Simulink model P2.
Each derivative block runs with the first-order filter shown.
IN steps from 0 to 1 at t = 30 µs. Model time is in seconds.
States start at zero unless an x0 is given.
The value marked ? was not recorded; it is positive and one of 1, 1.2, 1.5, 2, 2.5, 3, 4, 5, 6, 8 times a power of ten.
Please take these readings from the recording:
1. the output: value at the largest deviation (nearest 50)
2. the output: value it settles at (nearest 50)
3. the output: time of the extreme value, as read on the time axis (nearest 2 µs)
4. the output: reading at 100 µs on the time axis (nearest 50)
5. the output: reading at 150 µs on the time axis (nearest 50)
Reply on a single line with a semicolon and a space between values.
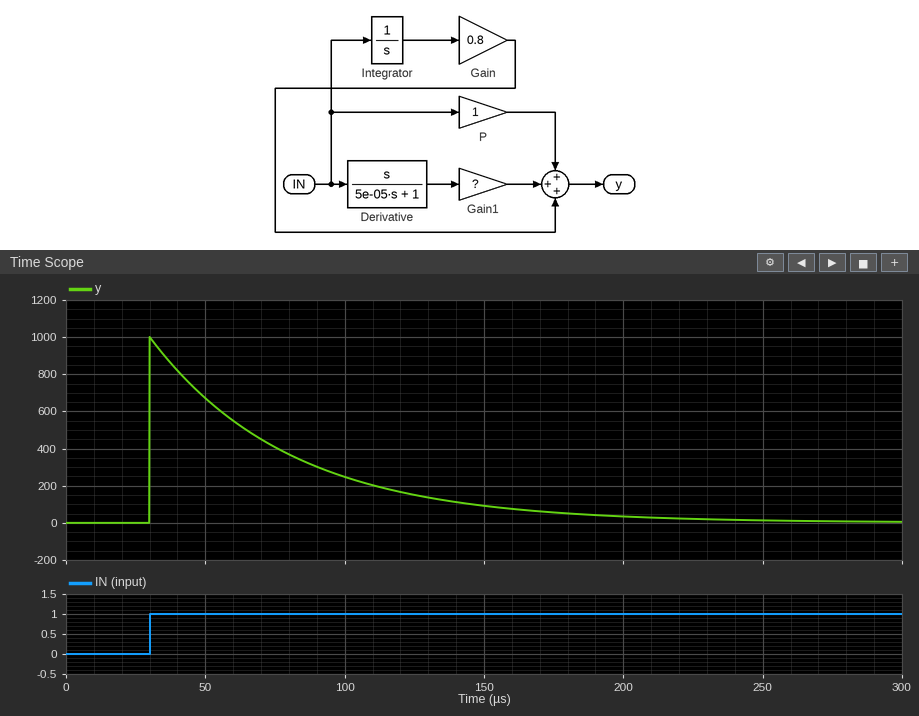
1000; 0; 30 µs; 250; 100
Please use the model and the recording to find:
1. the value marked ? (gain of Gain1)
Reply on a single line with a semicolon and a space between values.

0.05
